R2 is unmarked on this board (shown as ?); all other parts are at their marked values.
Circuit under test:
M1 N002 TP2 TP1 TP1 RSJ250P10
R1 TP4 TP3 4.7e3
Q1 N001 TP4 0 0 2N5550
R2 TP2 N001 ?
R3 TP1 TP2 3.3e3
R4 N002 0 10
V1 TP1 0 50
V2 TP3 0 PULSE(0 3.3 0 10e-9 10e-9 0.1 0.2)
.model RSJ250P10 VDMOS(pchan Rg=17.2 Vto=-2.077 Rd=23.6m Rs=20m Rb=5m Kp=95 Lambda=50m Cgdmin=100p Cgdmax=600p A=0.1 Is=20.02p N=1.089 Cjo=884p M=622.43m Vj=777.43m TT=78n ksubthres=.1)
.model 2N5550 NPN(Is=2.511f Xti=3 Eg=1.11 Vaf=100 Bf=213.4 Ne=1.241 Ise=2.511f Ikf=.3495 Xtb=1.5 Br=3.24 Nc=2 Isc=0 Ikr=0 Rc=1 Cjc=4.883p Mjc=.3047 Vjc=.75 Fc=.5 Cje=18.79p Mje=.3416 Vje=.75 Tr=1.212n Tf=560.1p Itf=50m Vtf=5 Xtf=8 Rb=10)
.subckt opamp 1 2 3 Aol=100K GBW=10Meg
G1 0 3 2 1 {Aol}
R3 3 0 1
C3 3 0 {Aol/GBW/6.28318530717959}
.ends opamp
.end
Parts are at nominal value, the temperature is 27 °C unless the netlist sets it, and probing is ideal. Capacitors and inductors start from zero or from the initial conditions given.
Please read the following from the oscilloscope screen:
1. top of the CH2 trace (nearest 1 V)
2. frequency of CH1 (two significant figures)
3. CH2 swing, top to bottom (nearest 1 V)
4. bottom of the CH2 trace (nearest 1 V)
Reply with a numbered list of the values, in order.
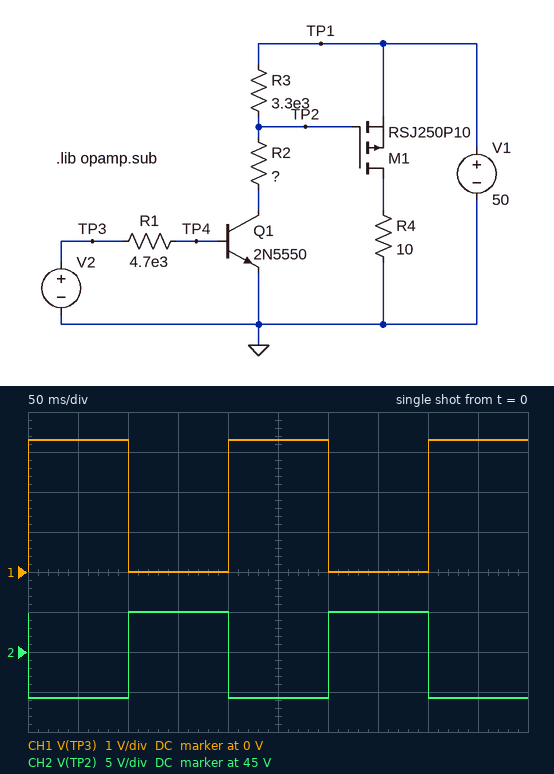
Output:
1. 50 V
2. 5.0 Hz
3. 11 V
4. 39 V
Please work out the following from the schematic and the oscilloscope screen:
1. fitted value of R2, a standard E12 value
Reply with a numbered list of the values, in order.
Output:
1. 12 kΩ
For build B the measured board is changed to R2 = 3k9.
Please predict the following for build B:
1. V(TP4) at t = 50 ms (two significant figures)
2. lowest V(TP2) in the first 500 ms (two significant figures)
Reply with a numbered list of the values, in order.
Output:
1. 750 mV
2. 27 V
